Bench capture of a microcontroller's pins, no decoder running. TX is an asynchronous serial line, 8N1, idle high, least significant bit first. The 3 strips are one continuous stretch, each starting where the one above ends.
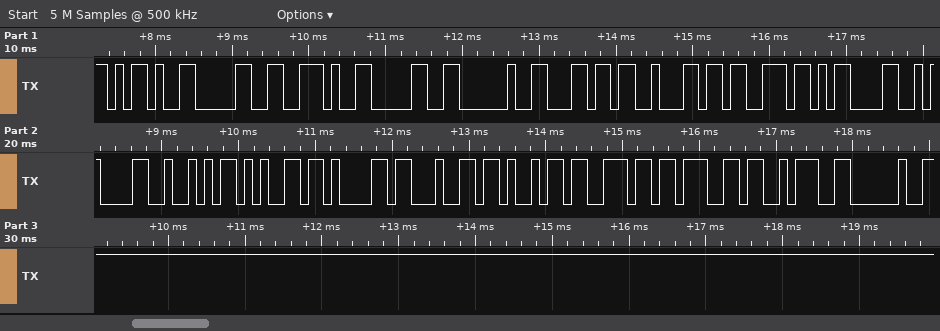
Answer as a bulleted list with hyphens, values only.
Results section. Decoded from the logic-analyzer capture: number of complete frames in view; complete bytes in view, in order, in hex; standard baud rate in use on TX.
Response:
- 19
- 0x2D 0x30 0x2E 0x30 0x20 0x6C 0x62 0x73 0x0D 0x0A 0x52 0x65 0x61 0x64 0x69 0x6E 0x67 0x3A 0x20
- 9600 baud
